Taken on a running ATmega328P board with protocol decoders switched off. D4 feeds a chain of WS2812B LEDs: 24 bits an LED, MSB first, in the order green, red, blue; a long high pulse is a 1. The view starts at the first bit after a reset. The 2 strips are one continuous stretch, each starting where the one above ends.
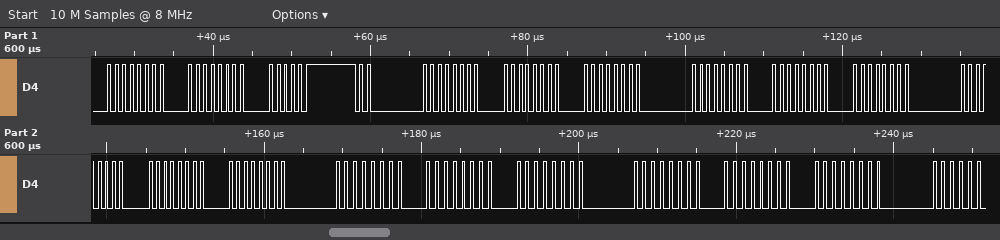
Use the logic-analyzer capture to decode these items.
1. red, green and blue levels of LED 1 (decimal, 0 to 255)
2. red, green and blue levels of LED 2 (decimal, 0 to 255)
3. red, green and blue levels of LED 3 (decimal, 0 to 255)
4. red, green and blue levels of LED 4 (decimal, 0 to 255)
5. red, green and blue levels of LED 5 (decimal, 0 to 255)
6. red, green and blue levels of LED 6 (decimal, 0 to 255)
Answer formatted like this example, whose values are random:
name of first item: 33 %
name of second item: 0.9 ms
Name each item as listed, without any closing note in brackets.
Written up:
red, green and blue levels of LED 1: 0, 0, 4
red, green and blue levels of LED 2: 0, 0, 0
red, green and blue levels of LED 3: 0, 0, 0
red, green and blue levels of LED 4: 0, 0, 0
red, green and blue levels of LED 5: 0, 0, 0
red, green and blue levels of LED 6: 0, 0, 0
